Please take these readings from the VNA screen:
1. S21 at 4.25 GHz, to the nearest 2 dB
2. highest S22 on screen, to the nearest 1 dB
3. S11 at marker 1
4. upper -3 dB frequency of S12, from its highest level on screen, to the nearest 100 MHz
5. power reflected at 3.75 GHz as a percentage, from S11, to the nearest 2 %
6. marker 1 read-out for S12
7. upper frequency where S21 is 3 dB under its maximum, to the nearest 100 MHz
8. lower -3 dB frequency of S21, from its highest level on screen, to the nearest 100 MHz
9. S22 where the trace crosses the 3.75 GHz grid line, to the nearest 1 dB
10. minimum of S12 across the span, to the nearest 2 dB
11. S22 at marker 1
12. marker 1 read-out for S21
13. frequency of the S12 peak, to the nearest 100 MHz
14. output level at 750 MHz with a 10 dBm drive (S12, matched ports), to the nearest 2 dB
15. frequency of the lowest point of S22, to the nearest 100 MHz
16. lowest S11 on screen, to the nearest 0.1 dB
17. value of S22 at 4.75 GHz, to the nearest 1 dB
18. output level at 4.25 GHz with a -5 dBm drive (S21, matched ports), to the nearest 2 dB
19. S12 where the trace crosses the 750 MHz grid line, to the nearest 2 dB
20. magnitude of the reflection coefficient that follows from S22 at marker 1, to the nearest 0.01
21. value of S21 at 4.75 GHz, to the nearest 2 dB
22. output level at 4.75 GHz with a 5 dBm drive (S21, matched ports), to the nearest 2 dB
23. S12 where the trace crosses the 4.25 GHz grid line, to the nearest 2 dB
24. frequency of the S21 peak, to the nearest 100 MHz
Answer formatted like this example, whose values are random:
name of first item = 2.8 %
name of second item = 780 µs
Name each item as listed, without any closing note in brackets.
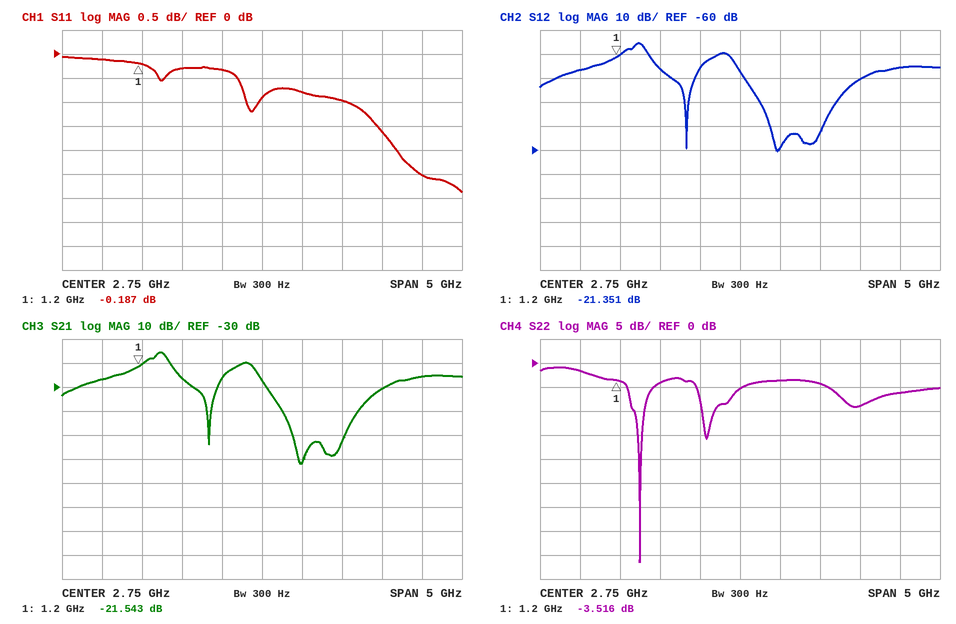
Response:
S21 at 4.25 GHz, to the nearest 2 dB = -30 dB
highest S22 on screen, to the nearest 1 dB = -1 dB
S11 at marker 1 = -0.187 dB
upper -3 dB frequency of S12, from its highest level on screen, to the nearest 100 MHz = 1.6 GHz
power reflected at 3.75 GHz as a percentage, from S11, to the nearest 2 % = 80 %
marker 1 read-out for S12 = -21.351 dB
upper frequency where S21 is 3 dB under its maximum, to the nearest 100 MHz = 1.6 GHz
lower -3 dB frequency of S21, from its highest level on screen, to the nearest 100 MHz = 1.3 GHz
S22 where the trace crosses the 3.75 GHz grid line, to the nearest 1 dB = -4 dB
minimum of S12 across the span, to the nearest 2 dB = -60 dB
S22 at marker 1 = -3.516 dB
marker 1 read-out for S21 = -21.543 dB
frequency of the S12 peak, to the nearest 100 MHz = 1.5 GHz
output level at 750 MHz with a 10 dBm drive (S12, matched ports), to the nearest 2 dB = -16 dBm
frequency of the lowest point of S22, to the nearest 100 MHz = 1.5 GHz
lowest S11 on screen, to the nearest 0.1 dB = -2.9 dB
value of S22 at 4.75 GHz, to the nearest 1 dB = -6 dB
output level at 4.25 GHz with a -5 dBm drive (S21, matched ports), to the nearest 2 dB = -36 dBm
S12 where the trace crosses the 750 MHz grid line, to the nearest 2 dB = -26 dB
magnitude of the reflection coefficient that follows from S22 at marker 1, to the nearest 0.01 = 0.67
value of S21 at 4.75 GHz, to the nearest 2 dB = -26 dB
output level at 4.75 GHz with a 5 dBm drive (S21, matched ports), to the nearest 2 dB = -20 dBm
S12 where the trace crosses the 4.25 GHz grid line, to the nearest 2 dB = -30 dB
frequency of the S21 peak, to the nearest 100 MHz = 1.5 GHz
